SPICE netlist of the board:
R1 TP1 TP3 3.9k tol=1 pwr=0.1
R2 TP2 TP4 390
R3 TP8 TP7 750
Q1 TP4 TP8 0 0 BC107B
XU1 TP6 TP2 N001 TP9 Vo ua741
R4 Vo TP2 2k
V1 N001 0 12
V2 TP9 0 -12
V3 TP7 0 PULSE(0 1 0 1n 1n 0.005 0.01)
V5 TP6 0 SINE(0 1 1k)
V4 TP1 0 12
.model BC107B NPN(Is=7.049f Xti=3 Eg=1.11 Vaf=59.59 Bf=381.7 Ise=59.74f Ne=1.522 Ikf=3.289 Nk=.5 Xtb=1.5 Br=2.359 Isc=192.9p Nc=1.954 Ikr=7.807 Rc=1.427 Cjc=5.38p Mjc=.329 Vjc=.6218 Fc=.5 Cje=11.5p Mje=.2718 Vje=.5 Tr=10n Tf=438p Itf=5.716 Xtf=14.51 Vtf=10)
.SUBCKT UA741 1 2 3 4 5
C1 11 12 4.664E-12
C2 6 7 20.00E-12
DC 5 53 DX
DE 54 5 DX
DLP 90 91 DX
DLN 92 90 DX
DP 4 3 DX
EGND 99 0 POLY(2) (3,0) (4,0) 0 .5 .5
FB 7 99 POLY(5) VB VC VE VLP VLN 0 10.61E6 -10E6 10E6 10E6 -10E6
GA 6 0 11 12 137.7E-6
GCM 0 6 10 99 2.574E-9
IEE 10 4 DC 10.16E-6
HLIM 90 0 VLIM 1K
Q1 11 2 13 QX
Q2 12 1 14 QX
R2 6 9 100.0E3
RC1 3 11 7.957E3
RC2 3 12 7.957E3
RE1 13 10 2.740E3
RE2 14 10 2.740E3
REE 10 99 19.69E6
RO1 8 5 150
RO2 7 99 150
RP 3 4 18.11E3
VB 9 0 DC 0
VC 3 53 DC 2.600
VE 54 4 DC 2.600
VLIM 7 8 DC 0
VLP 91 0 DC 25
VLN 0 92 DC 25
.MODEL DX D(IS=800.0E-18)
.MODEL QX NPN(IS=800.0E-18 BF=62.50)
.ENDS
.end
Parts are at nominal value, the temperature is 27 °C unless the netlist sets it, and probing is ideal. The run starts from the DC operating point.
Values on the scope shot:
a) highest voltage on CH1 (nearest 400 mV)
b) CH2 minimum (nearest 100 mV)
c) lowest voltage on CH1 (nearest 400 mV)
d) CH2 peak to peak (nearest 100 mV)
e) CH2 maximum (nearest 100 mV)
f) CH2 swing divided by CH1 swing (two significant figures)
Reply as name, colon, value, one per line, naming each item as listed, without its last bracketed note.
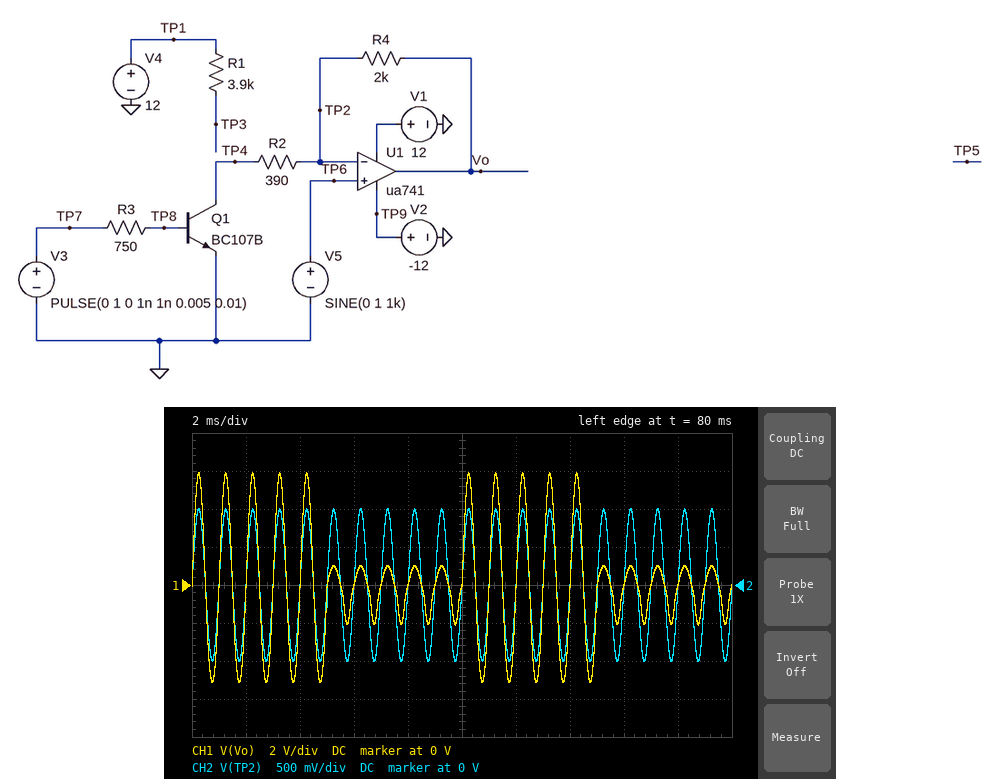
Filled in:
highest voltage on CH1: 6.0 V
CH2 minimum: -1.0 V
lowest voltage on CH1: -5.2 V
CH2 peak to peak: 2.0 V
CH2 maximum: 1.0 V
CH2 swing divided by CH1 swing: 0.18
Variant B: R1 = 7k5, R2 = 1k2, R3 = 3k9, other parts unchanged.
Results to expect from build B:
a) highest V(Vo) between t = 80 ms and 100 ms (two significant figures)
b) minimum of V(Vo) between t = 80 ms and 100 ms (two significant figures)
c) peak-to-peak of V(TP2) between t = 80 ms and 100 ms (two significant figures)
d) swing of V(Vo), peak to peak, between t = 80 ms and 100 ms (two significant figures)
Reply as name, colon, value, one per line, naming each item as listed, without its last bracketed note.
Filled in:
highest V(Vo) between t = 80 ms and 100 ms: 2.6 V
minimum of V(Vo) between t = 80 ms and 100 ms: -2.0 V
peak-to-peak of V(TP2) between t = 80 ms and 100 ms: 2.0 V
swing of V(Vo), peak to peak, between t = 80 ms and 100 ms: 4.6 V
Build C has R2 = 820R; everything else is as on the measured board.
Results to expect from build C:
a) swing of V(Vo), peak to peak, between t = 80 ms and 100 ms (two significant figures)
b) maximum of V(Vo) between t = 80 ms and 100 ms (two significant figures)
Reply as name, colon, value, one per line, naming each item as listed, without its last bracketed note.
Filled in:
swing of V(Vo), peak to peak, between t = 80 ms and 100 ms: 6.7 V
maximum of V(Vo) between t = 80 ms and 100 ms: 3.4 V
